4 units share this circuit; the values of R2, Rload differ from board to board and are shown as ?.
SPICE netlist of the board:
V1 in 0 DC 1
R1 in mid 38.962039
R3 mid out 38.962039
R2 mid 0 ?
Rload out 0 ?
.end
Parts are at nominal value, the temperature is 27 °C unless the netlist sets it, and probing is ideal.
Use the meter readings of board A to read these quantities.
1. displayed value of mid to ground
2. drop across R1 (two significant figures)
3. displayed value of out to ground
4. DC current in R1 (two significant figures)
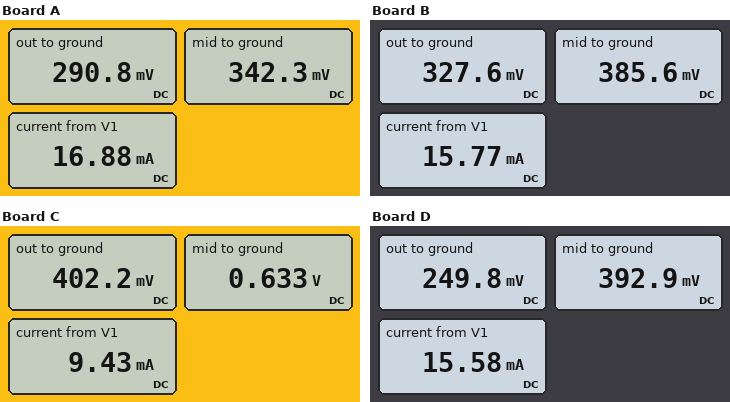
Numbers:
342.3 mV
660 mV
290.8 mV
17 mA
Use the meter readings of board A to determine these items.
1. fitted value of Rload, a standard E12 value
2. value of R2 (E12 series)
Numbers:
220 Ω
22 Ω
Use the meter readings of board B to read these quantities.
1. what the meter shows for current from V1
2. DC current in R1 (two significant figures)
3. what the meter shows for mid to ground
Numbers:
15.77 mA
16 mA
385.6 mV
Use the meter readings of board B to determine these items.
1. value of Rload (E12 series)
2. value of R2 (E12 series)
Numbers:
220 Ω
27 Ω
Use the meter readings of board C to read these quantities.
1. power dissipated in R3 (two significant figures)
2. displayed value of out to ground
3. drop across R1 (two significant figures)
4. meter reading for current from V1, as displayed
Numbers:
1.4 mW
402.2 mV
370 mV
9.43 mA
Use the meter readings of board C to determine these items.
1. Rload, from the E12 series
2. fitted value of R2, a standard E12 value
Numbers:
68 Ω
180 Ω
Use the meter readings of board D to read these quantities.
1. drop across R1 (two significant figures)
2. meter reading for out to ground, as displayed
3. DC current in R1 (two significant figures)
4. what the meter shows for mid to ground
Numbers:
610 mV
249.8 mV
16 mA
392.9 mV
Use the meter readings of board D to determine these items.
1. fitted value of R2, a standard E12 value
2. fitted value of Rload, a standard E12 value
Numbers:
33 Ω
68 Ω
